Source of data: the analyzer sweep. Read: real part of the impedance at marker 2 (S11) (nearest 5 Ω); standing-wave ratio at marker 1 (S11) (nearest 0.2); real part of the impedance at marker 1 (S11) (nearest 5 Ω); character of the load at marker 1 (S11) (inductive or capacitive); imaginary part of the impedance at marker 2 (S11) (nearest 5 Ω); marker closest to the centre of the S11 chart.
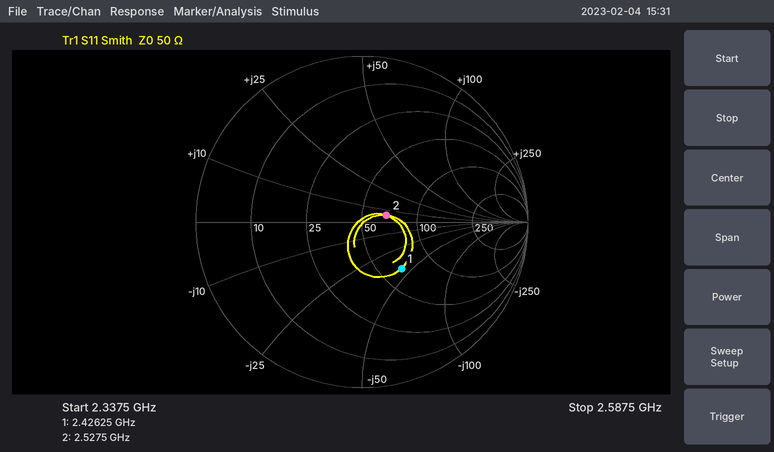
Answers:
65 Ω
2.2
65 Ω
capacitive
+5 Ω
marker 2
